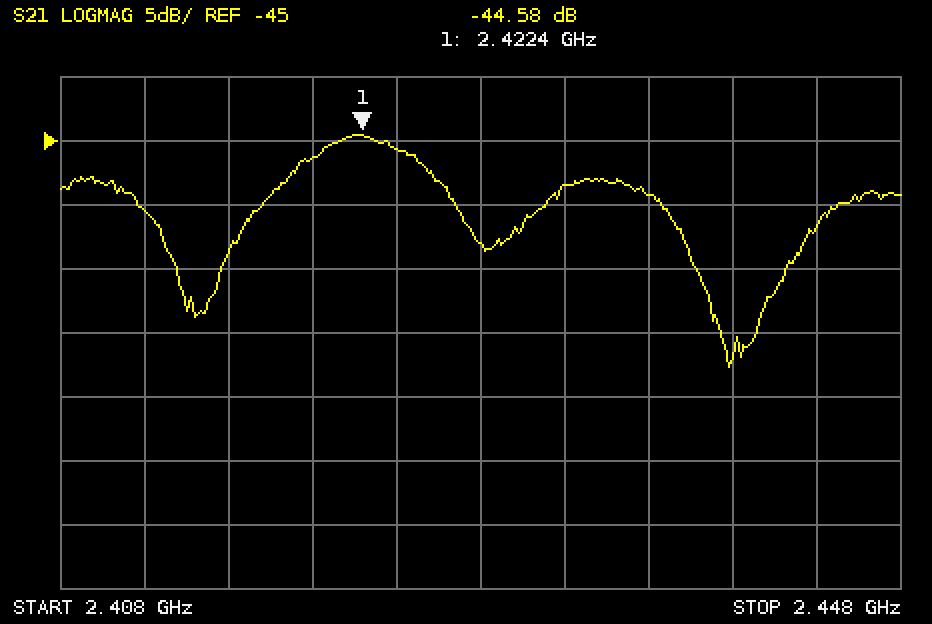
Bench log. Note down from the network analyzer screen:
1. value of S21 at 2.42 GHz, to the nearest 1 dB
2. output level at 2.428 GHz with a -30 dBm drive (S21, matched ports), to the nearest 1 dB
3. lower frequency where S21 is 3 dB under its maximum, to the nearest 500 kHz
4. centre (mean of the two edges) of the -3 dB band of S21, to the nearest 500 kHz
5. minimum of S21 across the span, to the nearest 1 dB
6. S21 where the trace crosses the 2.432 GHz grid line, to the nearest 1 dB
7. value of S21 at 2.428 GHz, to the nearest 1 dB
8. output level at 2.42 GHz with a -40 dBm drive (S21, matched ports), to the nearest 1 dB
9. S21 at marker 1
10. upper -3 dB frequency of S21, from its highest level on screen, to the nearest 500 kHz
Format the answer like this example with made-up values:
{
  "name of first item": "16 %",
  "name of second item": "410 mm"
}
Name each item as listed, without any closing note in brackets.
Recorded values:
{
  "value of S21 at 2.42 GHz, to the nearest 1 dB": "-46 dB",
  "output level at 2.428 GHz with a -30 dBm drive (S21, matched ports), to the nearest 1 dB": "-83 dBm",
  "lower frequency where S21 is 3 dB under its maximum, to the nearest 500 kHz": "2.4190 GHz",
  "centre (mean of the two edges) of the -3 dB band of S21, to the nearest 500 kHz": "2.4225 GHz",
  "minimum of S21 across the span, to the nearest 1 dB": "-63 dB",
  "S21 where the trace crosses the 2.432 GHz grid line, to the nearest 1 dB": "-48 dB",
  "value of S21 at 2.428 GHz, to the nearest 1 dB": "-53 dB",
  "output level at 2.42 GHz with a -40 dBm drive (S21, matched ports), to the nearest 1 dB": "-86 dBm",
  "S21 at marker 1": "-44.58 dB",
  "upper -3 dB frequency of S21, from its highest level on screen, to the nearest 500 kHz": "2.4255 GHz"
}
